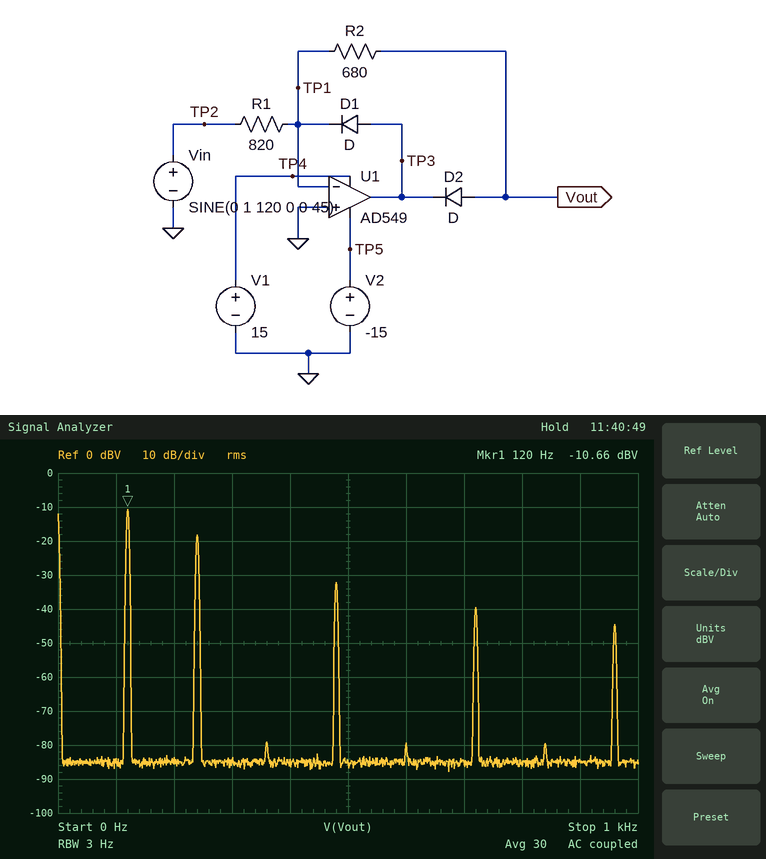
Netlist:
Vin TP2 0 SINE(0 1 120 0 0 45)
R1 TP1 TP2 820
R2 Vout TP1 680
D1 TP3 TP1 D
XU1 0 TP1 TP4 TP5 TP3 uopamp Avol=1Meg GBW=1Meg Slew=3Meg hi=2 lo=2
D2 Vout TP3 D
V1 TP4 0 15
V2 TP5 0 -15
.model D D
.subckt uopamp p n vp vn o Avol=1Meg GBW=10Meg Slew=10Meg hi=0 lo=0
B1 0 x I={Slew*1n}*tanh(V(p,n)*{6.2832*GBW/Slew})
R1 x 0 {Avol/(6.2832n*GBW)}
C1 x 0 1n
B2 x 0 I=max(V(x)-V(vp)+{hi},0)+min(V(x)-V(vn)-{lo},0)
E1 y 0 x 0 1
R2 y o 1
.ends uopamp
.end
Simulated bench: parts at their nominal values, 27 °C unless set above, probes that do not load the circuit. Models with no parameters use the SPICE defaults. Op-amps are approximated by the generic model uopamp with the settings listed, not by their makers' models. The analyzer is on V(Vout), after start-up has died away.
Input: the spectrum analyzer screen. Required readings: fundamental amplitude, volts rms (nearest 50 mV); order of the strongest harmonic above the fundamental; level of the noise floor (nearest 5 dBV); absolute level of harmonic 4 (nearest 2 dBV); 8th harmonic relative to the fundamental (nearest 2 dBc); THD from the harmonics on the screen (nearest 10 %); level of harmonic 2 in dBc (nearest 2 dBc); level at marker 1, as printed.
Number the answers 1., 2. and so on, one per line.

1. 300 mV
2. 2
3. -85 dBV
4. -32 dBV
5. -34 dBc
6. 40 %
7. -8 dBc
8. -10.66 dBV
